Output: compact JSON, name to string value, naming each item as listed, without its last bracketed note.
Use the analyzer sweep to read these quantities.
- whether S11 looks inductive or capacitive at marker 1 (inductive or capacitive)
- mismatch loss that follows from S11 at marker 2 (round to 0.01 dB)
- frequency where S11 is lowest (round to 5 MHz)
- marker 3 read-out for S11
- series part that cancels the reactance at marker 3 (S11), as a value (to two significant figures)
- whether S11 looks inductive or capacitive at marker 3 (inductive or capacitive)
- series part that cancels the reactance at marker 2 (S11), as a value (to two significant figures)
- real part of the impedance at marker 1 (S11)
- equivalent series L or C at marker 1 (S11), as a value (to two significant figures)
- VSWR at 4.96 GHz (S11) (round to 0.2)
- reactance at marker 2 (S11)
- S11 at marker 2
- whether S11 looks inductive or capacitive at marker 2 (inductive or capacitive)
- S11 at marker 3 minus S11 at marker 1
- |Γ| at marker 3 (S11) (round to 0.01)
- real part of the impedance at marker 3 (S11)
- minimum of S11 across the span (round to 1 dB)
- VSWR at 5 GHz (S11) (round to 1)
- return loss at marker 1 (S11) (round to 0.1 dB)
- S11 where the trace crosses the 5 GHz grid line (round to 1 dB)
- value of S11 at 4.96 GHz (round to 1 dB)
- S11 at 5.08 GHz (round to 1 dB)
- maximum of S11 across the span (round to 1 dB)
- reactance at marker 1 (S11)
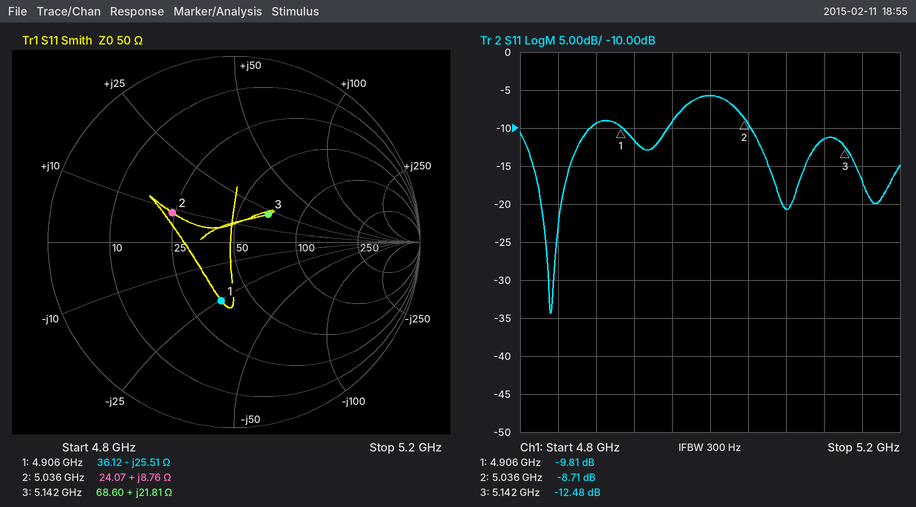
{"whether S11 looks inductive or capacitive at marker 1": "capacitive", "mismatch loss that follows from S11 at marker 2": "0.63 dB", "frequency where S11 is lowest": "4.830 GHz", "marker 3 read-out for S11": "-12.48 dB", "series part that cancels the reactance at marker 3 (S11), as a value": "1.4 pF", "whether S11 looks inductive or capacitive at marker 3": "inductive", "series part that cancels the reactance at marker 2 (S11), as a value": "3.6 pF", "real part of the impedance at marker 1": "36.12 Ω", "equivalent series L or C at marker 1 (S11), as a value": "1.3 pF", "VSWR at 4.96 GHz (S11)": "2.0", "reactance at marker 2": "+8.76 Ω", "S11 at marker 2": "-8.71 dB", "whether S11 looks inductive or capacitive at marker 2": "inductive", "S11 at marker 3 minus S11 at marker 1": "-2.67 dB", "|Γ| at marker 3 (S11)": "0.24", "real part of the impedance at marker 3": "68.60 Ω", "minimum of S11 across the span": "-34 dB", "VSWR at 5 GHz (S11)": "3", "return loss at marker 1 (S11)": "9.8 dB", "S11 where the trace crosses the 5 GHz grid line": "-6 dB", "value of S11 at 4.96 GHz": "-9 dB", "S11 at 5.08 GHz": "-21 dB", "maximum of S11 across the span": "-6 dB", "reactance at marker 1": "-25.51 Ω"}
